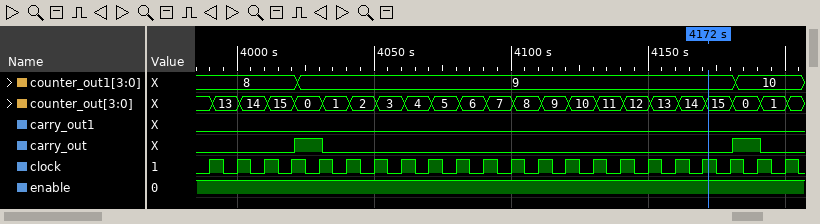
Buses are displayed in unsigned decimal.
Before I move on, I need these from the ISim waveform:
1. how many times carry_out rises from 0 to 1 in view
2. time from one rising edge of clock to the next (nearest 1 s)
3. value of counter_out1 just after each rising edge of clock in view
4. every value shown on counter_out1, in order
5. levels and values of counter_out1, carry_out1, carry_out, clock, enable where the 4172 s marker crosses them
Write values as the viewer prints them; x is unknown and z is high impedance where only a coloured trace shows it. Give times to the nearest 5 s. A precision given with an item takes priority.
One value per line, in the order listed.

2
10 s
8, 8, 8, 8, 9, 9, 9, 9, 9, 9, 9, 9, 9, 9, 9, 9, 9, 9, 9, 9, 10, 10
8, 9, 10
counter_out1=9, carry_out1=0, carry_out=0, clock=1, enable=1
